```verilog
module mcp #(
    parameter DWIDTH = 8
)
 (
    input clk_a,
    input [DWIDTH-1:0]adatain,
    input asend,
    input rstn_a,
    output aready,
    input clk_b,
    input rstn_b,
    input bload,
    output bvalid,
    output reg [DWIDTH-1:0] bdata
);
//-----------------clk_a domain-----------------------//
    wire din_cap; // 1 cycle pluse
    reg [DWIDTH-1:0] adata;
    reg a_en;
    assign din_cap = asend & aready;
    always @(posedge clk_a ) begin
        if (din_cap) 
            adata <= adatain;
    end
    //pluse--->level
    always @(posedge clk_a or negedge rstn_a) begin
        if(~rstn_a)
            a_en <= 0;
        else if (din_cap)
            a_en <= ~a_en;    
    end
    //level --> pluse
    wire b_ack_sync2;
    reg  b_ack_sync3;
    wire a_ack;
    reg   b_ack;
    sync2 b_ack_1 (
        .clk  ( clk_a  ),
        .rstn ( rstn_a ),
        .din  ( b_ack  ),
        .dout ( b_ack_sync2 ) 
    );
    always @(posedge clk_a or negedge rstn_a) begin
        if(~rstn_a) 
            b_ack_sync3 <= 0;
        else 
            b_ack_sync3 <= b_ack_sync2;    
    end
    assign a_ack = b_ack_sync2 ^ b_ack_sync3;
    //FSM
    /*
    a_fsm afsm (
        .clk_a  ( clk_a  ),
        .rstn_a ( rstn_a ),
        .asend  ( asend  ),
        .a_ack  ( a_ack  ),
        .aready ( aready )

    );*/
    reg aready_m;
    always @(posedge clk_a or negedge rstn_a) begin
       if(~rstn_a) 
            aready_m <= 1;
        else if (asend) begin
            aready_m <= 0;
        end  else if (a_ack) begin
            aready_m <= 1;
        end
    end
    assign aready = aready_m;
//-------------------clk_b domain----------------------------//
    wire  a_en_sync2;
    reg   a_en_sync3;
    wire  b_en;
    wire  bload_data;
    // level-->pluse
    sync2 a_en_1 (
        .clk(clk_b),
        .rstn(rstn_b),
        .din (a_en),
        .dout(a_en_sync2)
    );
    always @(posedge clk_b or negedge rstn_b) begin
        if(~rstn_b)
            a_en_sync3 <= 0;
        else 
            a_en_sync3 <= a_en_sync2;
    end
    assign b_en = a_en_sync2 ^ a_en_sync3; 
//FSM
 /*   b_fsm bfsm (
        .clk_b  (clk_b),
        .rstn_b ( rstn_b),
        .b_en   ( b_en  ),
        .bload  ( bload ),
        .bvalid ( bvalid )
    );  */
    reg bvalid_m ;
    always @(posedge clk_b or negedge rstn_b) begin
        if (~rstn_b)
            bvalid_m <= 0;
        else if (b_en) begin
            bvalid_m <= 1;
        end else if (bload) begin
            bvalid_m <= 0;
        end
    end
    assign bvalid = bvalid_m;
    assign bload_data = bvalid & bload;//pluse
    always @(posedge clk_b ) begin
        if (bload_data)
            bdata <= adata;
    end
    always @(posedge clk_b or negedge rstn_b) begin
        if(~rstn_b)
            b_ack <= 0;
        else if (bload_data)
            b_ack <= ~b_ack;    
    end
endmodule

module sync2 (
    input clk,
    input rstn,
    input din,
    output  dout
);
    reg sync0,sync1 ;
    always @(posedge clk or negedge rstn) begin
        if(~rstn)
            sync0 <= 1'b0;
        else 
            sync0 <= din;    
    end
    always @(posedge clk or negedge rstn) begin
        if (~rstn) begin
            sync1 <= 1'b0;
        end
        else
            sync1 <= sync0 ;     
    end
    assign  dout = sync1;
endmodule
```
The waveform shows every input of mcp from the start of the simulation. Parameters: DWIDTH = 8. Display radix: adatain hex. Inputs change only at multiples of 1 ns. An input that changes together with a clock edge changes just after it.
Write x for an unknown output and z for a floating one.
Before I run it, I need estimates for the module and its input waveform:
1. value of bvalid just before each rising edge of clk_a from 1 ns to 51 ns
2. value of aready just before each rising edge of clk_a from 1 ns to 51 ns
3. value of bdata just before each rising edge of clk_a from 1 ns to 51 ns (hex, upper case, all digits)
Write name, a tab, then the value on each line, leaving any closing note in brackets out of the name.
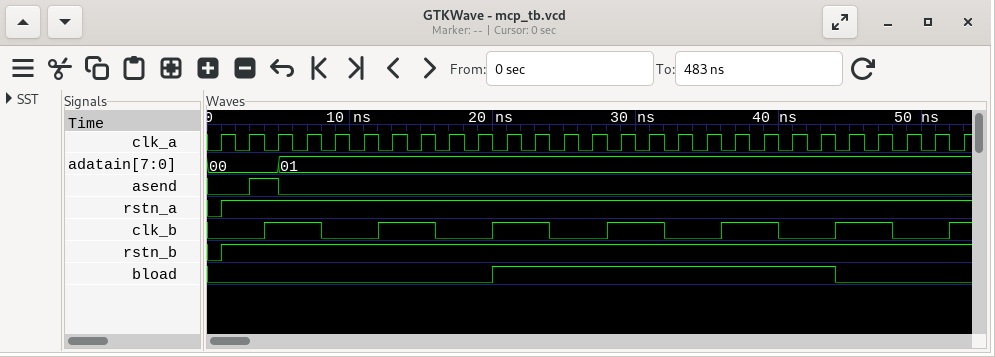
value of bvalid just before each rising edge of clk_a from 1 ns to 51 ns	0 0 0 0 0 0 0 0 0 0 0 0 0 0 1 1 1 1 0 0 0 0 0 0 0 0
value of aready just before each rising edge of clk_a from 1 ns to 51 ns	1 1 1 0 0 0 0 0 0 0 0 0 0 0 0 0 0 0 0 0 0 1 1 1 1 1
value of bdata just before each rising edge of clk_a from 1 ns to 51 ns	x, x, x, x, x, x, x, x, x, x, x, x, x, x, x, x, x, x, 00, 00, 00, 00, 00, 00, 00, 00
